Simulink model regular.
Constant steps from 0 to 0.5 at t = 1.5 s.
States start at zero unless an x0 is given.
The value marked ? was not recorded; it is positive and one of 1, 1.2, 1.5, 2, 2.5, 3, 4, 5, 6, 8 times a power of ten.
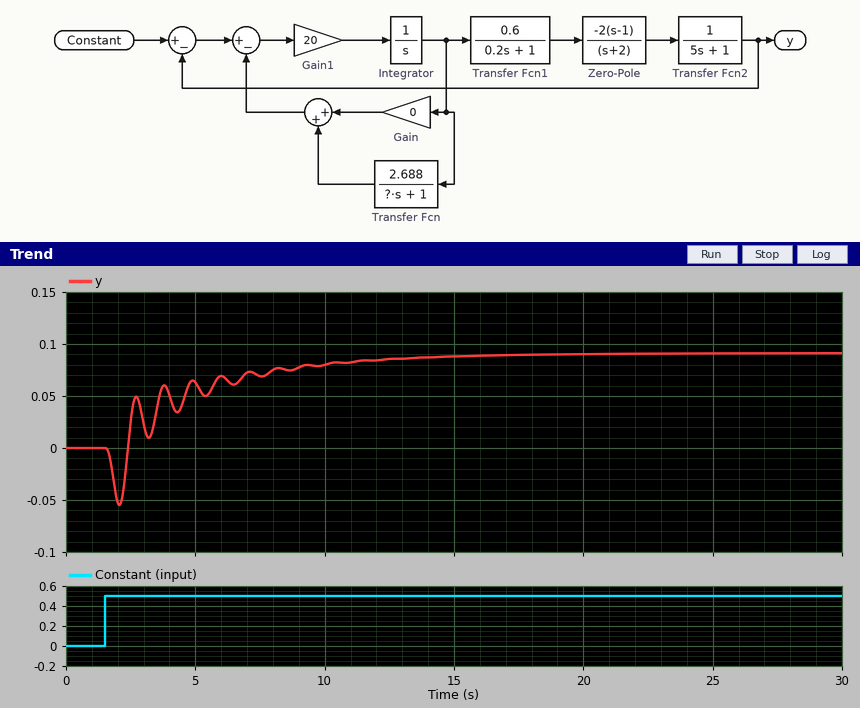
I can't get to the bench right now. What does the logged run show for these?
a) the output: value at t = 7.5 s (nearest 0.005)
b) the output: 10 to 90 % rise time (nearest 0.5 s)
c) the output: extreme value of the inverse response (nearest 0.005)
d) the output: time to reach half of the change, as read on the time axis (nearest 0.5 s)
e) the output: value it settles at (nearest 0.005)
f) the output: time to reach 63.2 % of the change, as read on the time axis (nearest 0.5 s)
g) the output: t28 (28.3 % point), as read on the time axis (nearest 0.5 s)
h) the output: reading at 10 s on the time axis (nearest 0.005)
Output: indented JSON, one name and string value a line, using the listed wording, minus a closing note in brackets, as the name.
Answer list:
{
  "the output: value at t = 7.5 s": "0.070",
  "the output: 10 to 90 % rise time": "8.0 s",
  "the output: extreme value of the inverse response": "-0.055",
  "the output: time to reach half of the change, as read on the time axis": "2.5 s",
  "the output: value it settles at": "0.090",
  "the output: time to reach 63.2 % of the change, as read on the time axis": "3.5 s",
  "the output: t28 (28.3 % point), as read on the time axis": "2.5 s",
  "the output: reading at 10 s on the time axis": "0.080"
}
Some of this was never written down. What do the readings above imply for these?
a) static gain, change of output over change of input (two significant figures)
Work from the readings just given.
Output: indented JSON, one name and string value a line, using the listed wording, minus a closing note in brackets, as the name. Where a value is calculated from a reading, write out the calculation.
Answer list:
{
  "static gain, change of output over change of input": "(0.09 - 0) / (0.5 - 0) = 0.18"
}
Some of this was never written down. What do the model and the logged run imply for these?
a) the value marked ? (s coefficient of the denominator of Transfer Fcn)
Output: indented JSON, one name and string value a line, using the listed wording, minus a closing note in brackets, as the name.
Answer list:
{
  "the value marked ?": "1.5"
}
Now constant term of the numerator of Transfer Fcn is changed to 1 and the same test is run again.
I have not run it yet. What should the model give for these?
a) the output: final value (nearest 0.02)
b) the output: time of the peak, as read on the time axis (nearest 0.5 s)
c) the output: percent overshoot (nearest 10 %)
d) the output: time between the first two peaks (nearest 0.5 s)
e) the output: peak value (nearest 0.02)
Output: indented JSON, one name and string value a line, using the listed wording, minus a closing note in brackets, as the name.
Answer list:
{
  "the output: final value": "0.18",
  "the output: time of the peak, as read on the time axis": "3.5 s",
  "the output: percent overshoot": "30 %",
  "the output: time between the first two peaks": "2.0 s",
  "the output: peak value": "0.24"
}
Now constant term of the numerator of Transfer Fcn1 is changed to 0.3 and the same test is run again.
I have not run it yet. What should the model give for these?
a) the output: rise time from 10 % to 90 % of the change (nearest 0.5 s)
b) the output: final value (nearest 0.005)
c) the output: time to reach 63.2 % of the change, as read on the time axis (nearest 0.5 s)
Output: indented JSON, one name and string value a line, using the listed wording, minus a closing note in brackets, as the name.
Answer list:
{
  "the output: rise time from 10 % to 90 % of the change": "9.0 s",
  "the output: final value": "0.050",
  "the output: time to reach 63.2 % of the change, as read on the time axis": "4.5 s"
}
